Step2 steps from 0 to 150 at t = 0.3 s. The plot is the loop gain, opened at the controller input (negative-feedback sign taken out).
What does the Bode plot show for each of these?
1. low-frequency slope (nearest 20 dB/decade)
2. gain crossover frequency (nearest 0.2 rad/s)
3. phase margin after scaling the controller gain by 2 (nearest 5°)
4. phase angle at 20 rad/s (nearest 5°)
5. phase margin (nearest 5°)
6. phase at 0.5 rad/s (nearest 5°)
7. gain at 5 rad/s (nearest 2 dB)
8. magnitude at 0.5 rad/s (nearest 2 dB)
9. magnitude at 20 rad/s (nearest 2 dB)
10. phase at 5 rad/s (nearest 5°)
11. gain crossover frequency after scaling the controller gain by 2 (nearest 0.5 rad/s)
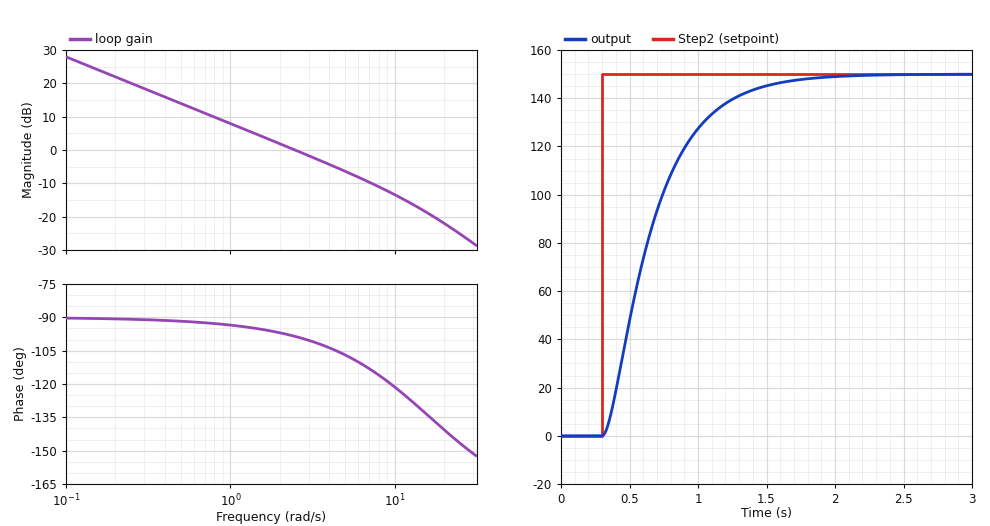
-20 dB/decade
2.4 rad/s
75°
-140°
80°
-90°
-6 dB
14 dB
-22 dB
-105°
5.0 rad/s
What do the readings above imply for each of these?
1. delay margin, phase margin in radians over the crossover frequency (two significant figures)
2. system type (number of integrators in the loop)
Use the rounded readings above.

0.58 s
1
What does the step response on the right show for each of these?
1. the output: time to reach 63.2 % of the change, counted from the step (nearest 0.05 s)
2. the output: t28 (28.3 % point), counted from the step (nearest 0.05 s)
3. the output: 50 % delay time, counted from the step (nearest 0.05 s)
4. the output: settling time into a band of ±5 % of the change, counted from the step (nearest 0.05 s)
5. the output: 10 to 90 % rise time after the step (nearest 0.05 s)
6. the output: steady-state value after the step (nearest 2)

0.40 s
0.20 s
0.30 s
1.05 s
0.75 s
150
